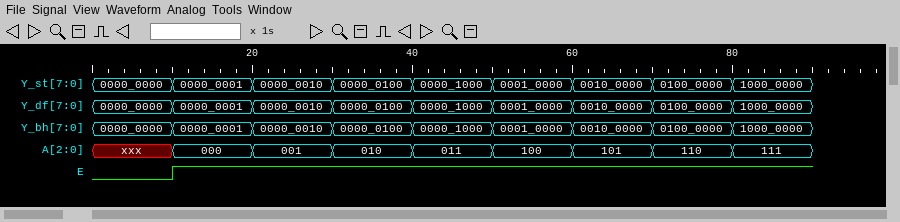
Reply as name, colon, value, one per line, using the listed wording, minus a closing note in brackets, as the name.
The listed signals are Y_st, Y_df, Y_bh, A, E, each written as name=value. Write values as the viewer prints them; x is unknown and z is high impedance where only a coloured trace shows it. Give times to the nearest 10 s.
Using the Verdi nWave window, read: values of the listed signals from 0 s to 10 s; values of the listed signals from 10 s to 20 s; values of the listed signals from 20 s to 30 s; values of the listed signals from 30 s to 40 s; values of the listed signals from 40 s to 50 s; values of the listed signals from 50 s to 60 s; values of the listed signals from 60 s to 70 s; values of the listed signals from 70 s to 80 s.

values of the listed signals from 0 s to 10 s: Y_st=0000_0000, Y_df=0000_0000, Y_bh=0000_0000, A=xxx, E=0
values of the listed signals from 10 s to 20 s: Y_st=0000_0001, Y_df=0000_0001, Y_bh=0000_0001, A=000, E=1
values of the listed signals from 20 s to 30 s: Y_st=0000_0010, Y_df=0000_0010, Y_bh=0000_0010, A=001, E=1
values of the listed signals from 30 s to 40 s: Y_st=0000_0100, Y_df=0000_0100, Y_bh=0000_0100, A=010, E=1
values of the listed signals from 40 s to 50 s: Y_st=0000_1000, Y_df=0000_1000, Y_bh=0000_1000, A=011, E=1
values of the listed signals from 50 s to 60 s: Y_st=0001_0000, Y_df=0001_0000, Y_bh=0001_0000, A=100, E=1
values of the listed signals from 60 s to 70 s: Y_st=0010_0000, Y_df=0010_0000, Y_bh=0010_0000, A=101, E=1
values of the listed signals from 70 s to 80 s: Y_st=0100_0000, Y_df=0100_0000, Y_bh=0100_0000, A=110, E=1
